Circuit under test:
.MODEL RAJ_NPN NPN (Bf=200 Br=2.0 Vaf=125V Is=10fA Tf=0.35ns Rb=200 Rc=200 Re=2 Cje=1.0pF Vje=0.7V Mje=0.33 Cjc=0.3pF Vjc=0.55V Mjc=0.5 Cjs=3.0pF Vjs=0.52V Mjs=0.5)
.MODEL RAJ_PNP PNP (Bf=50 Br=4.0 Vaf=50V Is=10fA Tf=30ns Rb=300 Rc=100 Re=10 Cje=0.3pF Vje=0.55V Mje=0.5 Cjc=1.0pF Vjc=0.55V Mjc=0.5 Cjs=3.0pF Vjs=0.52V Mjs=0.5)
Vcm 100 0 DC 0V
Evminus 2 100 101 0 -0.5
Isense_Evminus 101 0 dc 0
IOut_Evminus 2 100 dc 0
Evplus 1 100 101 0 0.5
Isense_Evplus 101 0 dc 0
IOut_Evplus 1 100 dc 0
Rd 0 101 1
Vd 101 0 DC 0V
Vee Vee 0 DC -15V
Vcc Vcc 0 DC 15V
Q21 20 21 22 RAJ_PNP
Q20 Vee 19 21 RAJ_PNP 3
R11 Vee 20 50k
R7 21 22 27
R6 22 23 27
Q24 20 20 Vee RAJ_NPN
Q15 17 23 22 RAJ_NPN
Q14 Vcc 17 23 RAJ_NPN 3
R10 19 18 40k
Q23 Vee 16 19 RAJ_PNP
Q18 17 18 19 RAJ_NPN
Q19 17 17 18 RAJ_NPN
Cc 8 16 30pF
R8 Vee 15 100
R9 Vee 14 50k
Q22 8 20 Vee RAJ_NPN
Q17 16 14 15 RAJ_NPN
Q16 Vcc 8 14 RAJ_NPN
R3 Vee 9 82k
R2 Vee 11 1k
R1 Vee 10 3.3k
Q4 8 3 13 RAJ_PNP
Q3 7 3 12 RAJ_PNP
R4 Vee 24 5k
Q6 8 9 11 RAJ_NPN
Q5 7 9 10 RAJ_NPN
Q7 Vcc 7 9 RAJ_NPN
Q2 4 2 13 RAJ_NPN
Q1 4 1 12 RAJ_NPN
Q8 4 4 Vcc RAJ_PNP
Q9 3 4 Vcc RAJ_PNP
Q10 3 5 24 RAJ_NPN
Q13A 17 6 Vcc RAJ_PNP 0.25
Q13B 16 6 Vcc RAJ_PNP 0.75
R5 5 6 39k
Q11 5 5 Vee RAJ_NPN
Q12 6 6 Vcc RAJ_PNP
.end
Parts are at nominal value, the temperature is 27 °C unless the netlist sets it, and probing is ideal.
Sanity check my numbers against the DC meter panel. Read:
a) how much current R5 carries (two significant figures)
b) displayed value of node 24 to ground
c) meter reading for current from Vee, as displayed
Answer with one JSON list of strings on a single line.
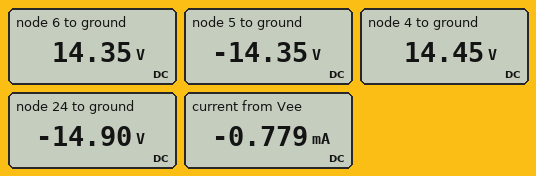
["740 µA", "-14.90 V", "-0.779 mA"]
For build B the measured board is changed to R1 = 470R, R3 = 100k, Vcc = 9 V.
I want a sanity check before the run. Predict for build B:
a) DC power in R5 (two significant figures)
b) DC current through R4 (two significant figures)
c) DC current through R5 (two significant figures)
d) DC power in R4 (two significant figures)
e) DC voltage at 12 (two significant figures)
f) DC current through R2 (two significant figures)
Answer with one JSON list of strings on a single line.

["13 mW", "19 µA", "580 µA", "1.7 µW", "-530 mV", "7.0 µA"]
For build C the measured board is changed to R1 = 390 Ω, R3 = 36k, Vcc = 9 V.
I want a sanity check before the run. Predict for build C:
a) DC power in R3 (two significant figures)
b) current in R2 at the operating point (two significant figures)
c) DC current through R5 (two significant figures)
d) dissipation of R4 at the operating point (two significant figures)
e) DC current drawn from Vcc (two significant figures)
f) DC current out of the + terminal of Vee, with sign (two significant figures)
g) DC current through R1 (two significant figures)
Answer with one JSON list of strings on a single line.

["7.9 µW", "6.9 µA", "580 µA", "1.7 µW", "1.8 mA", "-1.8 mA", "7.9 µA"]
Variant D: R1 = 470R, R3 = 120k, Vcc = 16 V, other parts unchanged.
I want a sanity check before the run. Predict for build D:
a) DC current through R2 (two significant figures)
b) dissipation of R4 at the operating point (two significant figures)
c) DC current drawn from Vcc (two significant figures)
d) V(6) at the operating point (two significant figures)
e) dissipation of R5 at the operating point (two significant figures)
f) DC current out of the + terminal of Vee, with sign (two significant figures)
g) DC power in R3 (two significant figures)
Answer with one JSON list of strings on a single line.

["6.7 µA", "2.0 µW", "2.2 mA", "15 V", "23 mW", "-2.2 mA", "2.4 µW"]
